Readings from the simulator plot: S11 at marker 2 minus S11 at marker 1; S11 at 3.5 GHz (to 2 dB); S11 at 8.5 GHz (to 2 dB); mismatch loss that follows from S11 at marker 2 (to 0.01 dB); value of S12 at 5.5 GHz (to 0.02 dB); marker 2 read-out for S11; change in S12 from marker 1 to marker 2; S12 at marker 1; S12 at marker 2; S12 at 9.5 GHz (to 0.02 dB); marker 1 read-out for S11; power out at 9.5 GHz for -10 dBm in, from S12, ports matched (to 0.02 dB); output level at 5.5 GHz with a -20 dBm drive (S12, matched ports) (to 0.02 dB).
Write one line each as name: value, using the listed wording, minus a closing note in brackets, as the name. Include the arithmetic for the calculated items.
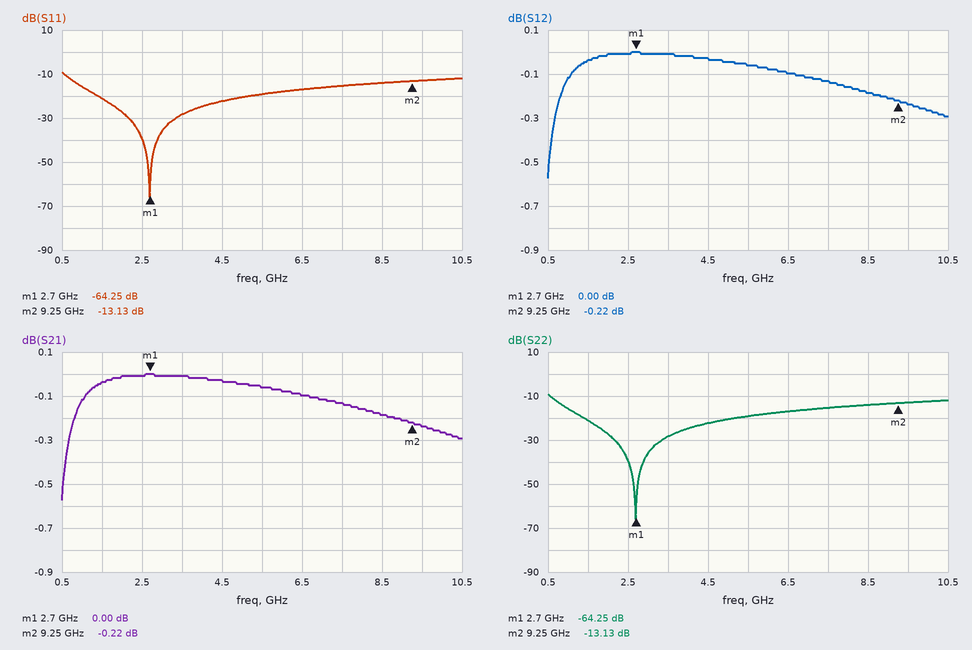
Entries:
S11 at marker 2 minus S11 at marker 1: -13.13 − (-64.25) = 51.12 dB
S11 at 3.5 GHz: -28 dB
S11 at 8.5 GHz: -14 dB
mismatch loss that follows from S11 at marker 2: −10 log10(1 − 10^(-13.13/10)) ≈ 0.22 dB
value of S12 at 5.5 GHz: -0.06 dB
marker 2 read-out for S11: -13.13 dB
change in S12 from marker 1 to marker 2: -0.22 − (0) = -0.22 dB
S12 at marker 1: 0.00 dB
S12 at marker 2: -0.22 dB
S12 at 9.5 GHz: -0.24 dB
marker 1 read-out for S11: -64.25 dB
power out at 9.5 GHz for -10 dBm in, from S12, ports matched: -10 dBm + (-0.24 dB) = -10.24 dBm
output level at 5.5 GHz with a -20 dBm drive (S12, matched ports): -20 dBm + (-0.06 dB) = -20.06 dBm
